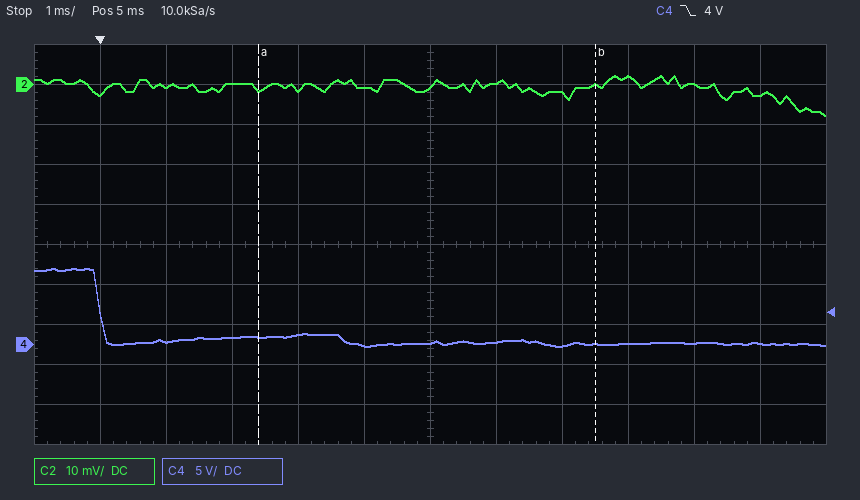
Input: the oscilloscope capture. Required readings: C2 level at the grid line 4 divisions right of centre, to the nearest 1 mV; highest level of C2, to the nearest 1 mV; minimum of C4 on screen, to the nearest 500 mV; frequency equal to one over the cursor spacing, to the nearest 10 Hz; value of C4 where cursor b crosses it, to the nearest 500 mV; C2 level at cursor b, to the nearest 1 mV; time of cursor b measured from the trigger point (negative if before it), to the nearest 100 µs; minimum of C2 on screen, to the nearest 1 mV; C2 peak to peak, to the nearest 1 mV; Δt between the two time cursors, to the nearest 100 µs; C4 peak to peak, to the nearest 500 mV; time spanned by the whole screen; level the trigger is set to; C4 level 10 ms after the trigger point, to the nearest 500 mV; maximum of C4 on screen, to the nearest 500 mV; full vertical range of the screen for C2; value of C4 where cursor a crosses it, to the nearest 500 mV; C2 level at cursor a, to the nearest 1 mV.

0 mV
2 mV
0.0 V
200 Hz
0.0 V
0 mV
+7.5 ms
-8 mV
10 mV
5.1 ms
9.5 V
12 ms
4 V
0.0 V
9.5 V
100 mV
1.0 V
-1 mV
